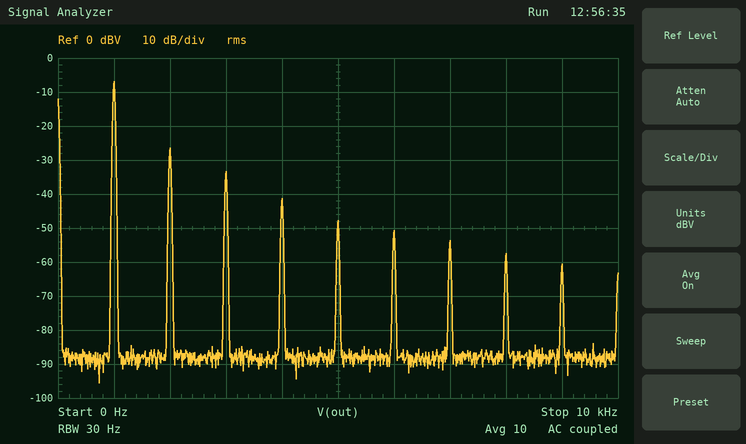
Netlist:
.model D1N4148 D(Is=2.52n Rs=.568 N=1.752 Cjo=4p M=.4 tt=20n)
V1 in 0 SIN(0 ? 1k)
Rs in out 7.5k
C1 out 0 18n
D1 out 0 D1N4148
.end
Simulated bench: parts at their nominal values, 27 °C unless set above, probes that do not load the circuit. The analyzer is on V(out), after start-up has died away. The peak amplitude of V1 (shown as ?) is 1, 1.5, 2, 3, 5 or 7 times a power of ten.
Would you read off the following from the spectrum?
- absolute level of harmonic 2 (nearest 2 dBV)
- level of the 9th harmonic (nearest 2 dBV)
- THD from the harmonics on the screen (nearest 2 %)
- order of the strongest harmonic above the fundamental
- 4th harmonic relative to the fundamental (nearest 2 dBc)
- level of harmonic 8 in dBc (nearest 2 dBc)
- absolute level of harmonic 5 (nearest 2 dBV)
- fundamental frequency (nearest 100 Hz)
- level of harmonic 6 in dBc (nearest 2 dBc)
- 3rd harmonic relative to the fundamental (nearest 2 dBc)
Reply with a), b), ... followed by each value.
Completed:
a) -26 dBV
b) -60 dBV
c) 12 %
d) 2
e) -34 dBc
f) -50 dBc
g) -48 dBV
h) 1.0 kHz
i) -44 dBc
j) -26 dBc
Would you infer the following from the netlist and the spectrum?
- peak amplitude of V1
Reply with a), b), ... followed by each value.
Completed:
a) 1 V
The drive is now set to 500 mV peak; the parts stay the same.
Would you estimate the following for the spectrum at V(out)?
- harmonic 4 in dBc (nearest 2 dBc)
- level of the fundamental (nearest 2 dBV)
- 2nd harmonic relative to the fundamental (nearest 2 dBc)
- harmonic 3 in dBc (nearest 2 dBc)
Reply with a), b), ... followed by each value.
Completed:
a) -48 dBc
b) -12 dBV
c) -36 dBc
d) -42 dBc
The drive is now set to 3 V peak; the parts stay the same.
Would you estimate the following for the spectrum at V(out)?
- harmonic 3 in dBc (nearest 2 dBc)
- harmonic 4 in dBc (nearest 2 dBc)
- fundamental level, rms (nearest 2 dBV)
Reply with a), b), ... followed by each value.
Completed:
a) -24 dBc
b) -32 dBc
c) 0 dBV
